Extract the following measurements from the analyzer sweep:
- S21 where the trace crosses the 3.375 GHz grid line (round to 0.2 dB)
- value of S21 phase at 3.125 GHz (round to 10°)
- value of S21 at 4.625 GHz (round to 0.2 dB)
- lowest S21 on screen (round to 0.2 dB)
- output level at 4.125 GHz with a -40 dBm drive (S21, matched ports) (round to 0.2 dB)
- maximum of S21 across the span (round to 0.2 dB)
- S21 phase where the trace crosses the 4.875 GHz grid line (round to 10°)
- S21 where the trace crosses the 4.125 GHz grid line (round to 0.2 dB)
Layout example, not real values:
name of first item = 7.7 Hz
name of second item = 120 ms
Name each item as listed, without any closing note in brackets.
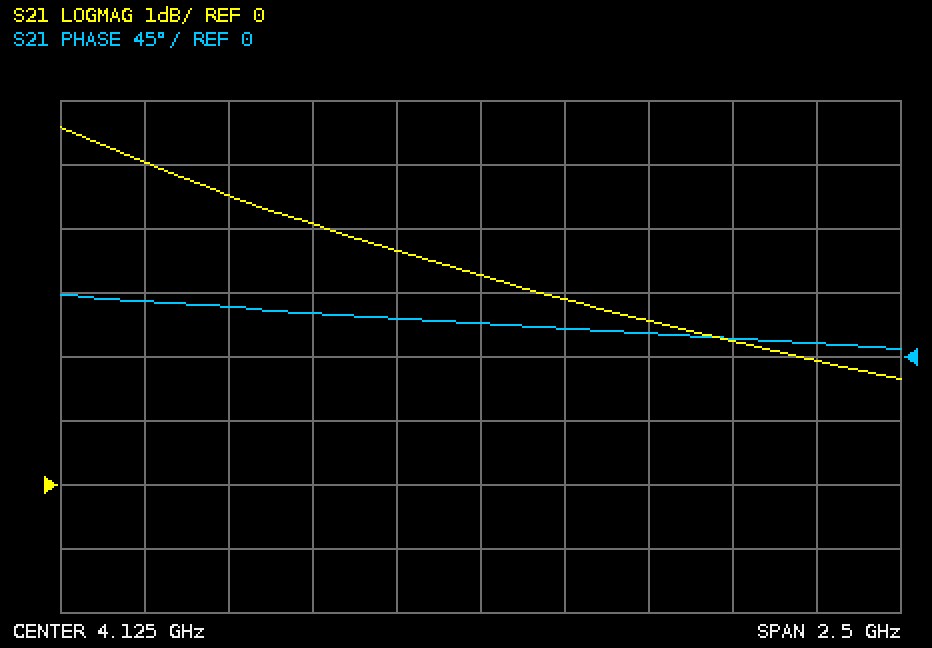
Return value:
S21 where the trace crosses the 3.375 GHz grid line = 4.6 dB
value of S21 phase at 3.125 GHz = 40°
value of S21 at 4.625 GHz = 2.6 dB
lowest S21 on screen = 1.6 dB
output level at 4.125 GHz with a -40 dBm drive (S21, matched ports) = -36.8 dBm
maximum of S21 across the span = 5.6 dB
S21 phase where the trace crosses the 4.875 GHz grid line = 10°
S21 where the trace crosses the 4.125 GHz grid line = 3.2 dB
